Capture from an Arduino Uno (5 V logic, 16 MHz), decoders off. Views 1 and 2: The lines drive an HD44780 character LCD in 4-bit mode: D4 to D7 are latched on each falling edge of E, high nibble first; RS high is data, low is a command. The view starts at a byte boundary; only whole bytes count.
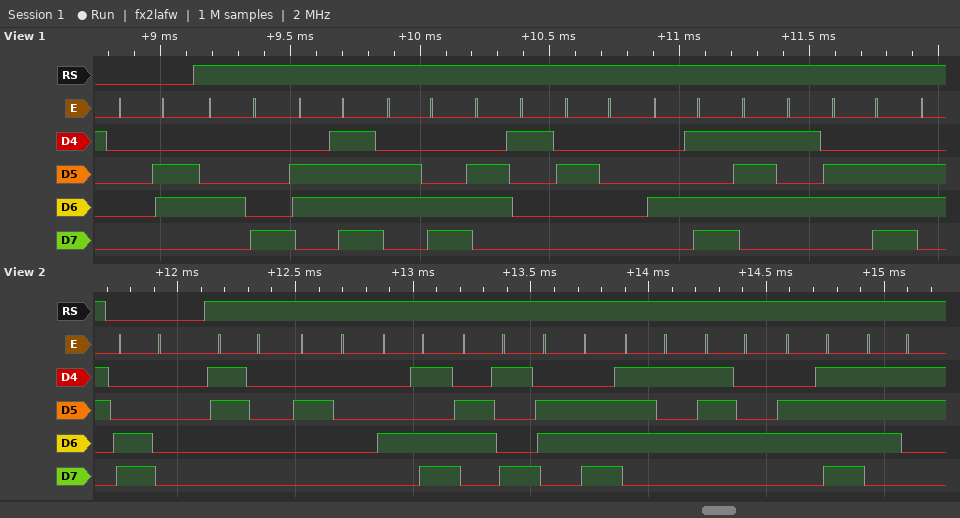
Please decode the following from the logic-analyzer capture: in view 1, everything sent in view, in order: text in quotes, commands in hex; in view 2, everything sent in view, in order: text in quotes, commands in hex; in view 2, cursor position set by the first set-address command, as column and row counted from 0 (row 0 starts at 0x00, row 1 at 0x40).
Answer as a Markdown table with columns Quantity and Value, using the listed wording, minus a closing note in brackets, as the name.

| Quantity | Value |
|---|---|
| in view 1, everything sent in view, in order: text in quotes, commands in hex | 0x06 "Hola Mun" |
| in view 2, everything sent in view, in order: text in quotes, commands in hex | 0xC0 "0 Minutos" |
| in view 2, cursor position set by the first set-address command, as column and row counted from 0 | column 0, row 1 |
